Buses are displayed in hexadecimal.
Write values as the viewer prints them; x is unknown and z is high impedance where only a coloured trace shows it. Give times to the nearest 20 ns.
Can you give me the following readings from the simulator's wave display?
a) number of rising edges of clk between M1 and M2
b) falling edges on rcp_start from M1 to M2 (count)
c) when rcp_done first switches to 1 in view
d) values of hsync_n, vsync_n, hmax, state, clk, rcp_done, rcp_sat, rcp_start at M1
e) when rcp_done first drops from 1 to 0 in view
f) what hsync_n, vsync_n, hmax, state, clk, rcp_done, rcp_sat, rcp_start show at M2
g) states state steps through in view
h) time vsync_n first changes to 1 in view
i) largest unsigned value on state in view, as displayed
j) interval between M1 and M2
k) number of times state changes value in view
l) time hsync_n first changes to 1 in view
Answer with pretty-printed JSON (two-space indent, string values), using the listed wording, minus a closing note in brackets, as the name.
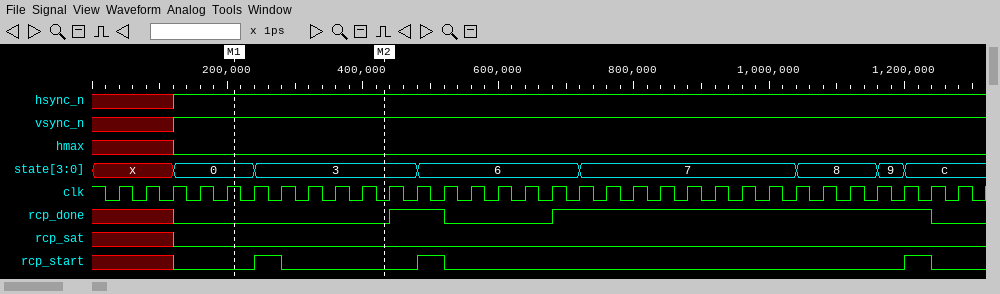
{
  "number of rising edges of clk between M1 and M2": "5",
  "falling edges on rcp_start from M1 to M2": "1",
  "when rcp_done first switches to 1 in view": "440 ns",
  "values of hsync_n, vsync_n, hmax, state, clk, rcp_done, rcp_sat, rcp_start at M1": "hsync_n=1, vsync_n=1, hmax=0, state=0, clk=1, rcp_done=0, rcp_sat=0, rcp_start=0",
  "when rcp_done first drops from 1 to 0 in view": "520 ns",
  "what hsync_n, vsync_n, hmax, state, clk, rcp_done, rcp_sat, rcp_start show at M2": "hsync_n=1, vsync_n=1, hmax=0, state=3, clk=0, rcp_done=0, rcp_sat=0, rcp_start=0",
  "states state steps through in view": "x, 0, 3, 6, 7, 8, 9, c",
  "time vsync_n first changes to 1 in view": "120 ns",
  "largest unsigned value on state in view, as displayed": "c",
  "interval between M1 and M2": "220 ns",
  "number of times state changes value in view": "7",
  "time hsync_n first changes to 1 in view": "120 ns"
}
